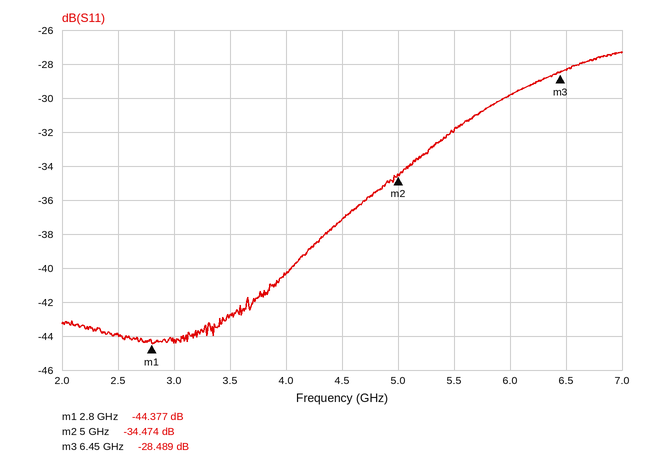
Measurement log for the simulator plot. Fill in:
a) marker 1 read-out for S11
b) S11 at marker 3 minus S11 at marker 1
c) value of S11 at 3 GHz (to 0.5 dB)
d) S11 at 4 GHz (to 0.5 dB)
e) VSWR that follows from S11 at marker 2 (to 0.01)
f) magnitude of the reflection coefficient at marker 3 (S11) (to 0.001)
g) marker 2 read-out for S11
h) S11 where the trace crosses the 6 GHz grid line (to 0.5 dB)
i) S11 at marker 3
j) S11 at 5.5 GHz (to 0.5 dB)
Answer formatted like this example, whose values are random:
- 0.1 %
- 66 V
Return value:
- -44.377 dB
- 15.888 dB
- -44.5 dB
- -40.5 dB
- 1.04
- 0.038
- -34.474 dB
- -30.0 dB
- -28.489 dB
- -32.0 dB
